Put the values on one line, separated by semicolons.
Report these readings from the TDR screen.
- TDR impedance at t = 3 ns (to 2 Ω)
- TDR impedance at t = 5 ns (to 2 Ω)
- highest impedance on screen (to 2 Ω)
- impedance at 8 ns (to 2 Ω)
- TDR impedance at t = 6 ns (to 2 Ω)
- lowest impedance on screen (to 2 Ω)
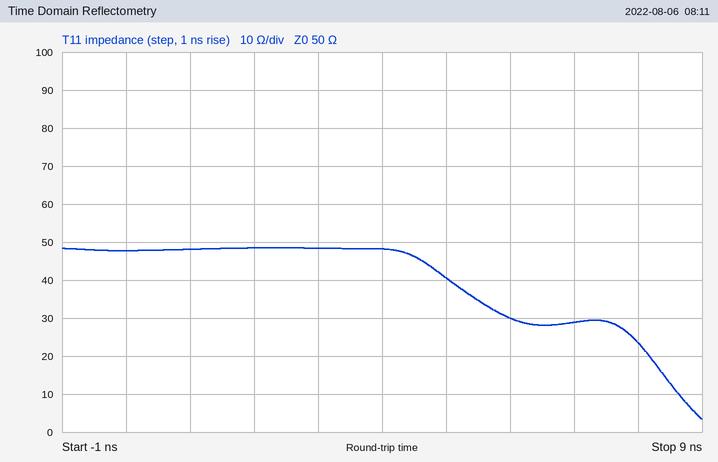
48 Ω; 40 Ω; 48 Ω; 24 Ω; 30 Ω; 4 Ω
